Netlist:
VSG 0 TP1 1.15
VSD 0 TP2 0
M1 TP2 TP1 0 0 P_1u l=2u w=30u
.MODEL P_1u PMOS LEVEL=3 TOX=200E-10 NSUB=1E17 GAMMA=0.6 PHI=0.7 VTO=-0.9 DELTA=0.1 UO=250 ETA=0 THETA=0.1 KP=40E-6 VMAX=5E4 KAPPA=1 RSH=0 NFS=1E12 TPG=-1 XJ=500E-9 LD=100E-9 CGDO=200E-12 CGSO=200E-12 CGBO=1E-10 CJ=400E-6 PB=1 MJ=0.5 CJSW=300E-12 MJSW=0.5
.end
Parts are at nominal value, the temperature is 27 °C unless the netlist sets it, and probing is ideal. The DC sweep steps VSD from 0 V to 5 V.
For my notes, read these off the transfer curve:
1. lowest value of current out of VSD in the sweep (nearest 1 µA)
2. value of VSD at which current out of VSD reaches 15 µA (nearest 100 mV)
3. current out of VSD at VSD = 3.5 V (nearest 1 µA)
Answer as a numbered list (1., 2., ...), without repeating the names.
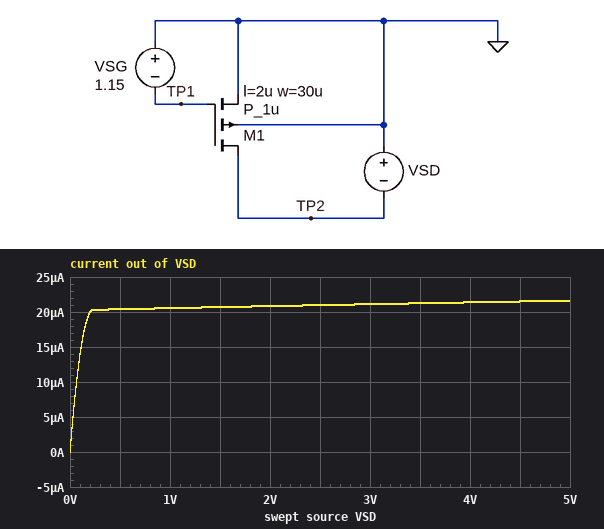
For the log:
1. 0 A
2. 100 mV
3. 21 µA
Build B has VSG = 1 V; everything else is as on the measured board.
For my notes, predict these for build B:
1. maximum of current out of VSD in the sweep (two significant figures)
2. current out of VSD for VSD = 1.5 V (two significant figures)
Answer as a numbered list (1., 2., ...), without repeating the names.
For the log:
1. 4.7 µA
2. 4.6 µA
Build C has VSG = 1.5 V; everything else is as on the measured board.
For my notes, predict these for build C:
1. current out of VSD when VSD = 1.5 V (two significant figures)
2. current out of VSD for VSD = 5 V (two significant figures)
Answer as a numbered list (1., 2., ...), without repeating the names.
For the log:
1. 96 µA
2. 100 µA
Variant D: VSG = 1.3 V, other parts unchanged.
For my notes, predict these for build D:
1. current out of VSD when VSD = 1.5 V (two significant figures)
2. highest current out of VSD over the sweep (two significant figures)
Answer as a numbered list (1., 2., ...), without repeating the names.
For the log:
1. 47 µA
2. 50 µA
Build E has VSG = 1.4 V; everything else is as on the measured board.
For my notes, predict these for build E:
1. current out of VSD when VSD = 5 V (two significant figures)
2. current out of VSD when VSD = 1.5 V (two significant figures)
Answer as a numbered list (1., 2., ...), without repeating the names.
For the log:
1. 74 µA
2. 70 µA
